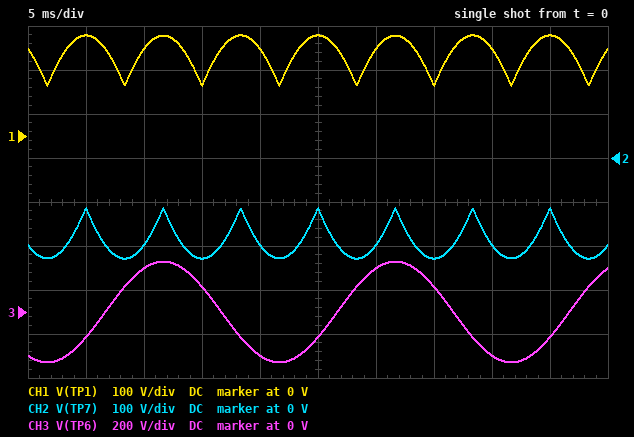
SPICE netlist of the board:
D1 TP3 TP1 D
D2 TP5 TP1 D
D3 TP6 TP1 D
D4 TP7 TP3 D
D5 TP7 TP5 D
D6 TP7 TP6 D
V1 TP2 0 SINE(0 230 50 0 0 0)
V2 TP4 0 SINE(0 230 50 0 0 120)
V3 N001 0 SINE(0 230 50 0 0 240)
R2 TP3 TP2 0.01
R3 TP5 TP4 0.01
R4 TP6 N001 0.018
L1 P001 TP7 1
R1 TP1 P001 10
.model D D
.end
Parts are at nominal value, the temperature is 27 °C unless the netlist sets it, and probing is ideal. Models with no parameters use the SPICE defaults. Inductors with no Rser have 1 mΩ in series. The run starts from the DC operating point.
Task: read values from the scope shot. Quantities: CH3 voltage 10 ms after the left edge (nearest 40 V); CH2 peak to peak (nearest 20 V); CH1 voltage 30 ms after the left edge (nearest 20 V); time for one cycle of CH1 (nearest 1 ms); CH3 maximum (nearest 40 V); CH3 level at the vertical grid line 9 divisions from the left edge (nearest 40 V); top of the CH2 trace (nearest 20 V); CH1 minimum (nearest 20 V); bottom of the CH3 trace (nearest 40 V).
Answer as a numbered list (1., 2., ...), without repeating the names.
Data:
1. 200 V
2. 120 V
3. 200 V
4. 7 ms
5. 240 V
6. -120 V
7. -120 V
8. 120 V
9. -240 V
